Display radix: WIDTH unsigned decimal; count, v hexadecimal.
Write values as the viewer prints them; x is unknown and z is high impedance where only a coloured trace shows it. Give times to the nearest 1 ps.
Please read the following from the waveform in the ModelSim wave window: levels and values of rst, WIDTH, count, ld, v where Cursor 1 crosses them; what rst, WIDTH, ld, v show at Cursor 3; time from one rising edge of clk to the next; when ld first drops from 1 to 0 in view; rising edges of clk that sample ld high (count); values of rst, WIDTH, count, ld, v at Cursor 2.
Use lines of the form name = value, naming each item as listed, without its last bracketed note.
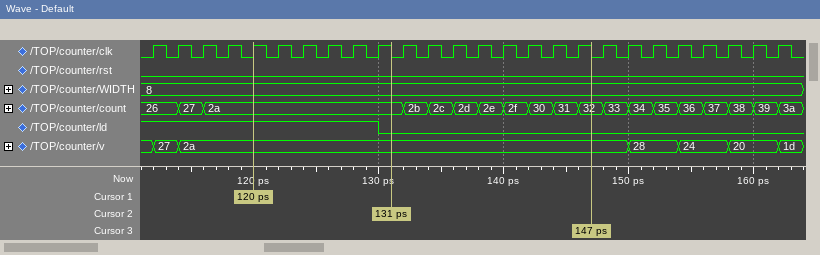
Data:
levels and values of rst, WIDTH, count, ld, v where Cursor 1 crosses them = rst=0, WIDTH=8, count=2a, ld=1, v=2a
what rst, WIDTH, ld, v show at Cursor 3 = rst=0, WIDTH=8, ld=0, v=2a
time from one rising edge of clk to the next = 2 ps
when ld first drops from 1 to 0 in view = 130 ps
rising edges of clk that sample ld high = 10
values of rst, WIDTH, count, ld, v at Cursor 2 = rst=0, WIDTH=8, count=2a, ld=0, v=2a
